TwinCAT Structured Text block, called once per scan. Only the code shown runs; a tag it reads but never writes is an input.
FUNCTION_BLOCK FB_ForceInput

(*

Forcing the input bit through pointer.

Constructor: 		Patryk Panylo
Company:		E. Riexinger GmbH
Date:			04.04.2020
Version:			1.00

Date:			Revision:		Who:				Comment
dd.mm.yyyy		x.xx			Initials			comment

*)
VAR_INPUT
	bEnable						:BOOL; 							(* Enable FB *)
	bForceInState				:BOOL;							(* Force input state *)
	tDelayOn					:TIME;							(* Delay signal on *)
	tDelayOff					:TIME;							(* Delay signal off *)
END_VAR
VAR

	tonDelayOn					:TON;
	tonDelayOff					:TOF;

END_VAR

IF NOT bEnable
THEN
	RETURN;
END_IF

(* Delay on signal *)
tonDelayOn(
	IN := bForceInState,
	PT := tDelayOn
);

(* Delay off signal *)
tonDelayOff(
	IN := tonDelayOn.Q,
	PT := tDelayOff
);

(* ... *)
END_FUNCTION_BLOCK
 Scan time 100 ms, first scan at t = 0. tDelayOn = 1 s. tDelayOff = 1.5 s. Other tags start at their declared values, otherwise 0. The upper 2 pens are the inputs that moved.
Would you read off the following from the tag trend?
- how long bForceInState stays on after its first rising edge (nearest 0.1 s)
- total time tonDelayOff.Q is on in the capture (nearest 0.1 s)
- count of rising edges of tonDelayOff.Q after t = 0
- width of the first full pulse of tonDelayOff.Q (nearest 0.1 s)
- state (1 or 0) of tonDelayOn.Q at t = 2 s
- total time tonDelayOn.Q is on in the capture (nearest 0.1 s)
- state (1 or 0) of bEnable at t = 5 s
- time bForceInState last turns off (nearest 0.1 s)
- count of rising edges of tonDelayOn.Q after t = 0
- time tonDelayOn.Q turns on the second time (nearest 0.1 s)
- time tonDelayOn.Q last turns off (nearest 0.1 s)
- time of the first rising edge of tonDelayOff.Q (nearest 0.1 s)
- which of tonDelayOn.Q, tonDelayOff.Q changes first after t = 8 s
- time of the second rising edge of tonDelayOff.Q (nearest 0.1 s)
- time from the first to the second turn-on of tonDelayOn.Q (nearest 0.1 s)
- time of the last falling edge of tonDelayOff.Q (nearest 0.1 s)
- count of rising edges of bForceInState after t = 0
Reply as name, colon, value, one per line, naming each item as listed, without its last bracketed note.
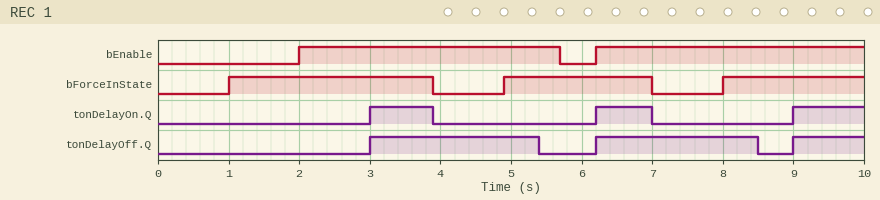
how long bForceInState stays on after its first rising edge: 2.9 s
total time tonDelayOff.Q is on in the capture: 5.7 s
count of rising edges of tonDelayOff.Q after t = 0: 3
width of the first full pulse of tonDelayOff.Q: 2.4 s
state (1 or 0) of tonDelayOn.Q at t = 2 s: 0
total time tonDelayOn.Q is on in the capture: 2.7 s
state (1 or 0) of bEnable at t = 5 s: 1
time bForceInState last turns off: 7.0 s
count of rising edges of tonDelayOn.Q after t = 0: 3
time tonDelayOn.Q turns on the second time: 6.2 s
time tonDelayOn.Q last turns off: 7.0 s
time of the first rising edge of tonDelayOff.Q: 3.0 s
which of tonDelayOn.Q, tonDelayOff.Q changes first after t = 8 s: tonDelayOff.Q
time of the second rising edge of tonDelayOff.Q: 6.2 s
time from the first to the second turn-on of tonDelayOn.Q: 3.2 s
time of the last falling edge of tonDelayOff.Q: 8.5 s
count of rising edges of bForceInState after t = 0: 3
